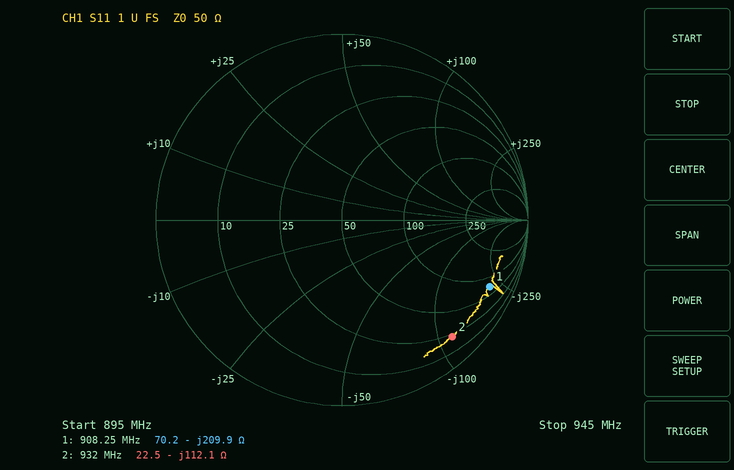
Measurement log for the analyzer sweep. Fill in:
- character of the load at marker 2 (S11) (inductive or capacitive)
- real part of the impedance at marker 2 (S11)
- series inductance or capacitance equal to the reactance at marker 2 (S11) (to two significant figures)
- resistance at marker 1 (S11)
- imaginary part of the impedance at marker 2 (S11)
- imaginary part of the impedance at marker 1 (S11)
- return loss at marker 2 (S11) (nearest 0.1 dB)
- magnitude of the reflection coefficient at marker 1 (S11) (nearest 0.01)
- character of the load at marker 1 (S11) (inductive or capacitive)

capacitive
22.5 Ω
1.5 pF
70.2 Ω
-112.1 Ω
-209.9 Ω
1.3 dB
0.87
capacitive
